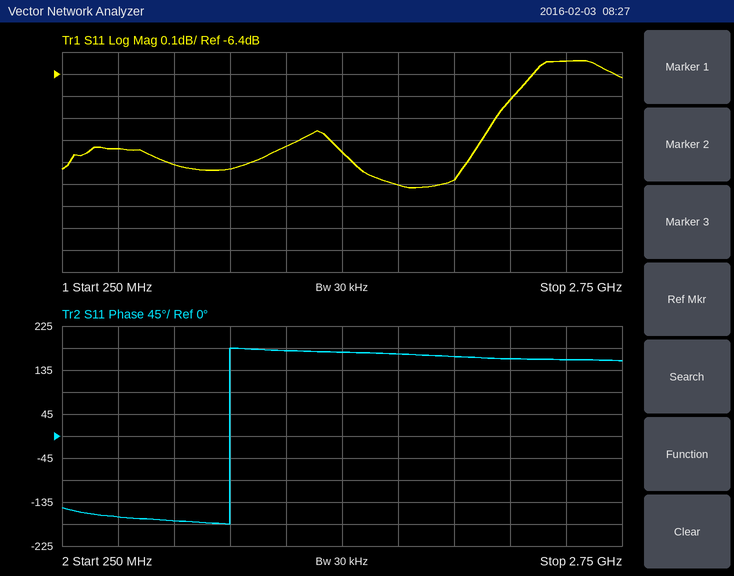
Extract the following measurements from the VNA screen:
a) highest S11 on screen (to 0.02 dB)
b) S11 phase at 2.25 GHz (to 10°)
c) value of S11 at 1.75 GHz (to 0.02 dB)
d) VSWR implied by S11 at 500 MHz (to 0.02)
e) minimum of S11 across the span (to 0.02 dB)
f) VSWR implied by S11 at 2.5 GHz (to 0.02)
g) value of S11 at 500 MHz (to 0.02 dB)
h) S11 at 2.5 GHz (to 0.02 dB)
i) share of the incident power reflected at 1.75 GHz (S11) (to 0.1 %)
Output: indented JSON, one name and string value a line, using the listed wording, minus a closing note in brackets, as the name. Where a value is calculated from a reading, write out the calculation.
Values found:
{
  "highest S11 on screen": "-6.34 dB",
  "S11 phase at 2.25 GHz": "160°",
  "value of S11 at 1.75 GHz": "-6.90 dB",
  "VSWR implied by S11 at 500 MHz": "|Γ| = 10^(-6.74/20) = 0.4603; VSWR = (1 + 0.4603)/(1 − 0.4603) ≈ 2.71, so 2.70 to the nearest 0.02",
  "minimum of S11 across the span": "-6.92 dB",
  "VSWR implied by S11 at 2.5 GHz": "|Γ| = 10^(-6.34/20) = 0.4819; VSWR = (1 + 0.4819)/(1 − 0.4819) ≈ 2.86",
  "value of S11 at 500 MHz": "-6.74 dB",
  "S11 at 2.5 GHz": "-6.34 dB",
  "share of the incident power reflected at 1.75 GHz (S11)": "10^(-6.9/10) ≈ 20.4 %"
}
